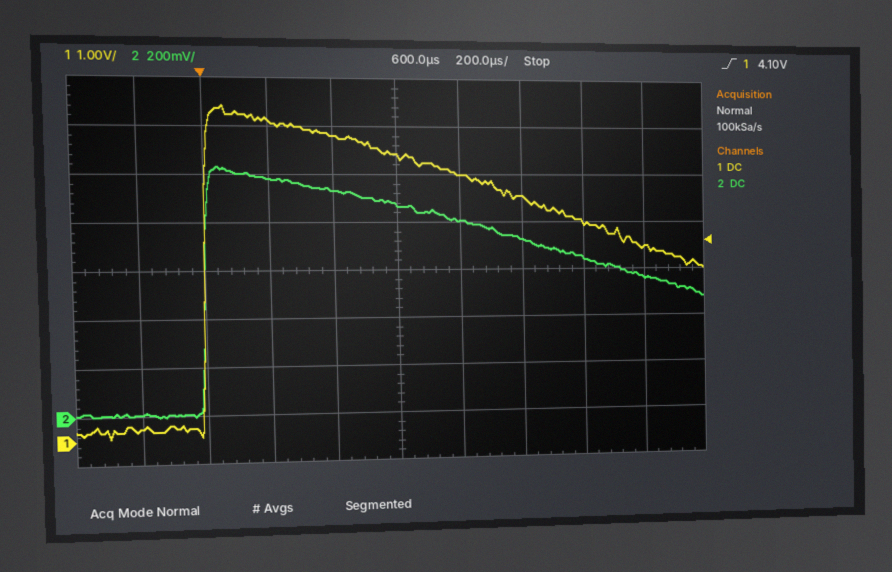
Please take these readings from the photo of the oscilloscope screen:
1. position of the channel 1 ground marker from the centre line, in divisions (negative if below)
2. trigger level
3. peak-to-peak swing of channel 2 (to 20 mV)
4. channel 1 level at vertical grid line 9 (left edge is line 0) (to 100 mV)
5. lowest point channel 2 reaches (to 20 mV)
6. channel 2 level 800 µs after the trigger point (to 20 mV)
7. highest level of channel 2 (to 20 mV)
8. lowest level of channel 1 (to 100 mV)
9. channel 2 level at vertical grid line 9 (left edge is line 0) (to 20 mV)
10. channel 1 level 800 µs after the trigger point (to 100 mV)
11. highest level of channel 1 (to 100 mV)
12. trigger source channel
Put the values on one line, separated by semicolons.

-3.5 div; 4.10 V; 1.04 V; 4.0 V; 0 mV; 800 mV; 1.04 V; 100 mV; 560 mV; 5.5 V; 6.9 V; channel 1
